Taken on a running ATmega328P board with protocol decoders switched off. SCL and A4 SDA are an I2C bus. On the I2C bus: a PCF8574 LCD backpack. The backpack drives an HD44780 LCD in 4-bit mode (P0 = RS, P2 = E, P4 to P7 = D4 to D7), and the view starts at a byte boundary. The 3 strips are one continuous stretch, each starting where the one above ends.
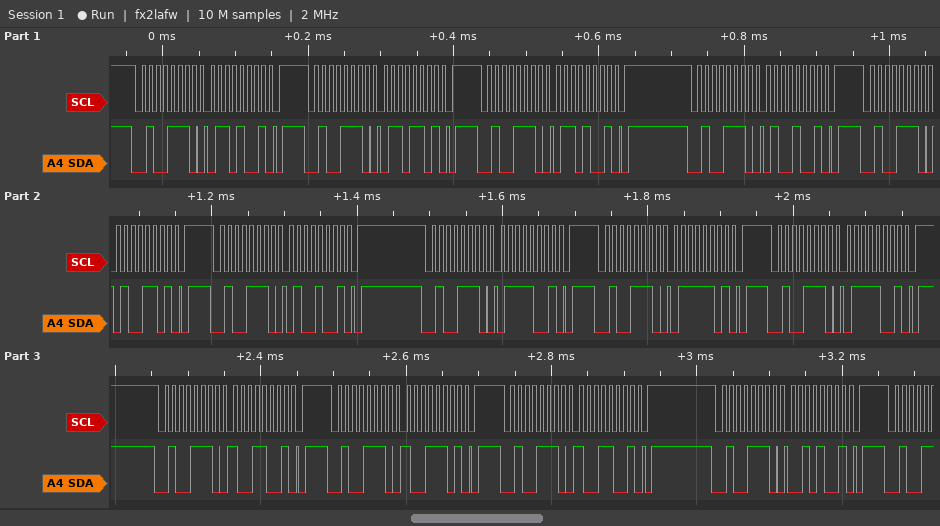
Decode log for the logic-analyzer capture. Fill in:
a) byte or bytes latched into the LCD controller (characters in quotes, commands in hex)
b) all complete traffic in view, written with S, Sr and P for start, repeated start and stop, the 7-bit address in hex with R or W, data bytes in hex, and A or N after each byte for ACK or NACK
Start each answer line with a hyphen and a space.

- 'd' 'y'
- S 27W A 69 A P S 27W A 6D A P S 27W A 69 A P S 27W A 49 A P S 27W A 4D A P S 27W A 49 A P S 27W A 79 A P S 27W A 7D A P S 27W A 79 A P S 27W A 99 A P S 27W A 9D A P S 27W A 99 A P S 27W A 29 A P
